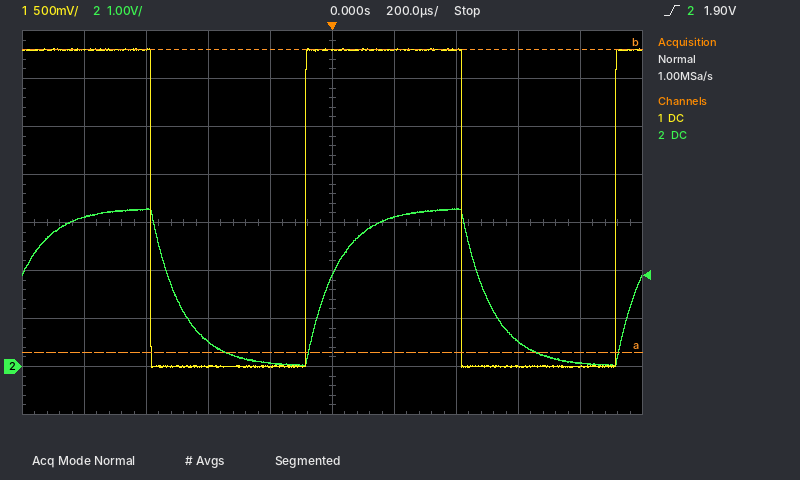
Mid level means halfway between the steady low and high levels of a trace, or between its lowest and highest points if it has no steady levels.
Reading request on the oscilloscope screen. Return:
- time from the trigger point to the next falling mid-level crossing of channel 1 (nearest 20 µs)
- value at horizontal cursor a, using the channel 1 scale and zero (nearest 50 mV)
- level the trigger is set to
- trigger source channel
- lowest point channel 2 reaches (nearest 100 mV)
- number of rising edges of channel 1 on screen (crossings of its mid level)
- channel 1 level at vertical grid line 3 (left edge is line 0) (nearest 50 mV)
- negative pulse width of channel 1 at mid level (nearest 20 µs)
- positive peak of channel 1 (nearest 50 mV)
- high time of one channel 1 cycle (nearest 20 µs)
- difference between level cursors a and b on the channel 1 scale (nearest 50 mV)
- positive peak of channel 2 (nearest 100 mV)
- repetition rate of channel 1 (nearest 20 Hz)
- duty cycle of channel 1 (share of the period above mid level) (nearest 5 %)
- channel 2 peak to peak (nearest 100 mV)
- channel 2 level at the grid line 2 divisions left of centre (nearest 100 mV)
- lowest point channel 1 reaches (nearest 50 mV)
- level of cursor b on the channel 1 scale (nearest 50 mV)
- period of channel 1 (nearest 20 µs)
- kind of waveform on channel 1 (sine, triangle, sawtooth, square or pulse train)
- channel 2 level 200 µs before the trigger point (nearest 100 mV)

420 µs
150 mV
1.90 V
channel 2
0.0 V
2
0 mV
500 µs
3.30 V
500 µs
3.15 V
3.3 V
1.00 kHz
50 %
3.3 V
500 mV
0 mV
3.30 V
1.00 ms
square
100 mV
